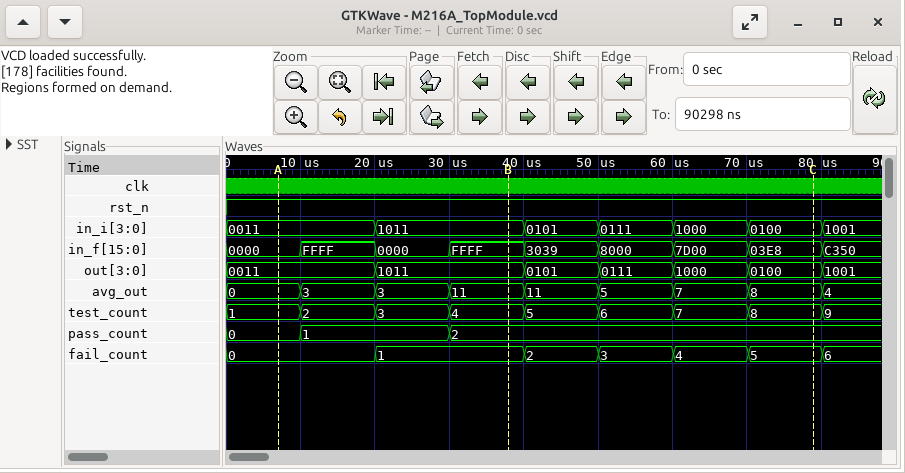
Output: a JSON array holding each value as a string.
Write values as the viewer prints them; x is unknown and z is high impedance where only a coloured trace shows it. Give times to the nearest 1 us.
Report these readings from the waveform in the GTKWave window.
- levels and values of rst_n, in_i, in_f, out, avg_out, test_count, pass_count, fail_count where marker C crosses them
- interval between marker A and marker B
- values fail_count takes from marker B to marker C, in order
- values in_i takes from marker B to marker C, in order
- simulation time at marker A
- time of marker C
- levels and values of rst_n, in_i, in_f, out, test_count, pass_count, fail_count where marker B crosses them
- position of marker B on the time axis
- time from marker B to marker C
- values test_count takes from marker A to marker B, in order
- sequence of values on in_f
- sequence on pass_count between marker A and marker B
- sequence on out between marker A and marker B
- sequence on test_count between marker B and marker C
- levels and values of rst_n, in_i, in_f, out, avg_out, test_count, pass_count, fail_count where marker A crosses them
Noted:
["rst_n=1, in_i=0100, in_f=03E8, out=0100, avg_out=8, test_count=8, pass_count=2, fail_count=5", "31 us", "1, 2, 3, 4, 5", "1011, 0101, 0111, 1000, 0100", "7 us", "79 us", "rst_n=1, in_i=1011, in_f=FFFF, out=1011, test_count=4, pass_count=2, fail_count=1", "38 us", "41 us", "1, 2, 3, 4", "0000, FFFF, 0000, FFFF, 3039, 8000, 7D00, 03E8, C350", "0, 1, 2", "0011, 1011", "4, 5, 6, 7, 8", "rst_n=1, in_i=0011, in_f=0000, out=0011, avg_out=0, test_count=1, pass_count=0, fail_count=0"]
